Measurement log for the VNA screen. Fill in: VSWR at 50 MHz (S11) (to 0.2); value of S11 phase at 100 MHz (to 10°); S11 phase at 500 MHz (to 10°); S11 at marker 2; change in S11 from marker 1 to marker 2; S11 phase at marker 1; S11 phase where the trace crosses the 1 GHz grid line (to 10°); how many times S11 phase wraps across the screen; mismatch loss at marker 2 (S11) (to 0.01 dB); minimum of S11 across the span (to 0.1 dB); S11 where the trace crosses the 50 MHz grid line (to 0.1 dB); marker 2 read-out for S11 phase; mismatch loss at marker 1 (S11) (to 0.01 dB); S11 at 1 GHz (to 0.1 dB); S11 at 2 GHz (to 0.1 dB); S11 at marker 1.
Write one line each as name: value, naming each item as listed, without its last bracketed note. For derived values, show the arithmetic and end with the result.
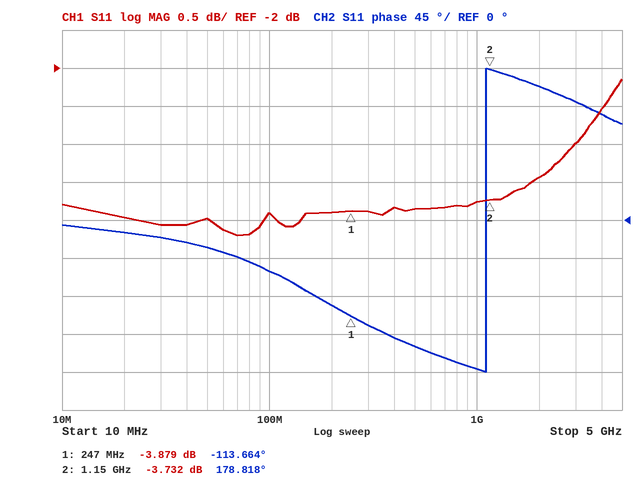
VSWR at 50 MHz (S11): |Γ| = 10^(-4/20) = 0.6310; VSWR = (1 + 0.6310)/(1 − 0.6310) ≈ 4.4
value of S11 phase at 100 MHz: -60°
S11 phase at 500 MHz: -150°
S11 at marker 2: -3.732 dB
change in S11 from marker 1 to marker 2: -3.732 − (-3.879) = 0.147 dB
S11 phase at marker 1: -113.664°
S11 phase where the trace crosses the 1 GHz grid line: -180°
how many times S11 phase wraps across the screen: 1
mismatch loss at marker 2 (S11): −10 log10(1 − 10^(-3.732/10)) ≈ 2.39 dB
minimum of S11 across the span: -4.2 dB
S11 where the trace crosses the 50 MHz grid line: -4.0 dB
marker 2 read-out for S11 phase: 178.818°
mismatch loss at marker 1 (S11): −10 log10(1 − 10^(-3.879/10)) ≈ 2.29 dB
S11 at 1 GHz: -3.8 dB
S11 at 2 GHz: -3.4 dB
S11 at marker 1: -3.879 dB
